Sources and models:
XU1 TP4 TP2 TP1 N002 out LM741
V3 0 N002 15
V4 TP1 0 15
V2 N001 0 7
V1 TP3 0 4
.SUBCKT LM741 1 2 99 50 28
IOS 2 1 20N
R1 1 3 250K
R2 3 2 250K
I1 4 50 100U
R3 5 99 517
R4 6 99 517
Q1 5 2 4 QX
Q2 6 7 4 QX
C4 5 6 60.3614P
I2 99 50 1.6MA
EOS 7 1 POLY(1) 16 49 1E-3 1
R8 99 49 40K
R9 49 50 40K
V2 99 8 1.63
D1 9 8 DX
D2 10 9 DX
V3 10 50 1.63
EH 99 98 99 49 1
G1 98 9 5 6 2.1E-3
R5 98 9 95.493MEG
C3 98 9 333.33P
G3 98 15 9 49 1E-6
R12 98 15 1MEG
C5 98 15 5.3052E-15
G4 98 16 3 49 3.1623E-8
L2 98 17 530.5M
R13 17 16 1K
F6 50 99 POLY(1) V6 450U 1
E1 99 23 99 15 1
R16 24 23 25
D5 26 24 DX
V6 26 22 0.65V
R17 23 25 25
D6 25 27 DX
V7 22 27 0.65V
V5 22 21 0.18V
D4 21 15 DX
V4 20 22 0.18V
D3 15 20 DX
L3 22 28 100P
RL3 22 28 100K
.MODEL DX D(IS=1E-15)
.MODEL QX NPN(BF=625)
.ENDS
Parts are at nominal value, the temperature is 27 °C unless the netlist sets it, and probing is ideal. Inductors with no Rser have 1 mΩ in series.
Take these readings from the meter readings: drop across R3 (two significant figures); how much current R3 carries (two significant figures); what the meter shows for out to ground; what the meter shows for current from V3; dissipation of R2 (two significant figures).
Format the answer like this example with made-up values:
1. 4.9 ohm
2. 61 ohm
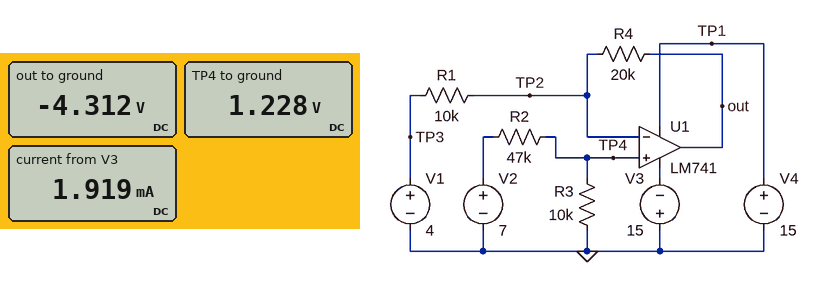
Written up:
1. 1.2 V
2. 120 µA
3. -4.312 V
4. 1.919 mA
5. 710 µW
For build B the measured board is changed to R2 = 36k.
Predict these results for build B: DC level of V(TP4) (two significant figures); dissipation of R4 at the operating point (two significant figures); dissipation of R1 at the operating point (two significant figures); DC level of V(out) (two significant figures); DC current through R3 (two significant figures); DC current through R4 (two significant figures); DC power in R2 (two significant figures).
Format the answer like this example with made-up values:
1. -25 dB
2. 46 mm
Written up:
1. 1.5 V
2. 1.2 mW
3. 610 µW
4. -3.4 V
5. 150 µA
6. 250 µA
7. 830 µW
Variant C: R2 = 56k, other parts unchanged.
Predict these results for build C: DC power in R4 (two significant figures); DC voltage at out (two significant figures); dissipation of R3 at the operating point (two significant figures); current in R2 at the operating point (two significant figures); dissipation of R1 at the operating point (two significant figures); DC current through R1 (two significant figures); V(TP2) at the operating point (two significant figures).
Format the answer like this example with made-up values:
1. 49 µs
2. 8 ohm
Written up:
1. 1.7 mW
2. -4.8 V
3. 110 µW
4. 110 µA
5. 860 µW
6. 290 µA
7. 1.1 V
